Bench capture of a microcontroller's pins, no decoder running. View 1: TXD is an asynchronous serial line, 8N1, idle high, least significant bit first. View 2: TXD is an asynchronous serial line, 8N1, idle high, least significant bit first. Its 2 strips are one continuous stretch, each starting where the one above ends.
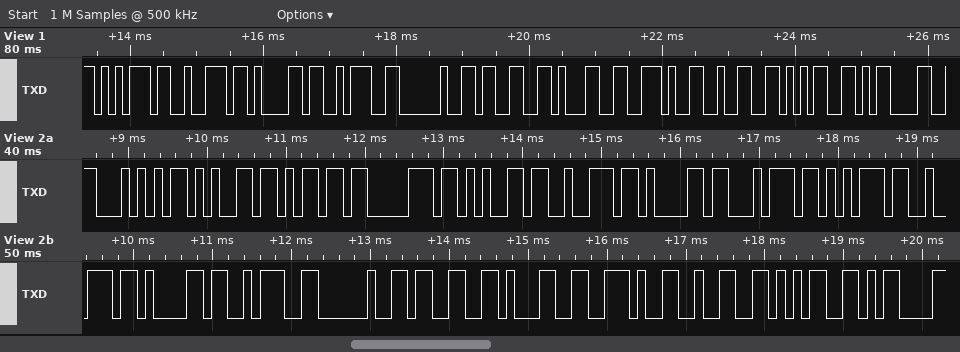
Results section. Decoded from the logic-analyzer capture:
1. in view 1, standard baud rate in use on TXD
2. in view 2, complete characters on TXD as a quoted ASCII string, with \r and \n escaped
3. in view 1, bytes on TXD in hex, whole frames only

9600 baud
"Temperatura: 31.25\r"
0x75 0x72 0x61 0x3A 0x20 0x33 0x31 0x2E 0x32 0x35 0x0D
